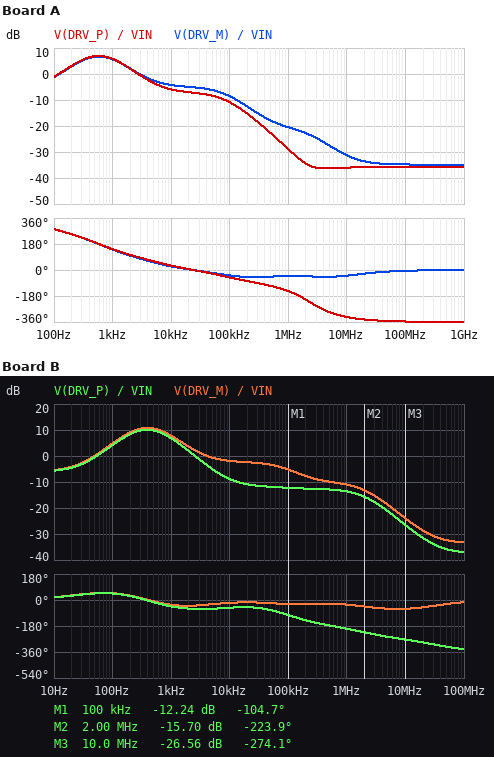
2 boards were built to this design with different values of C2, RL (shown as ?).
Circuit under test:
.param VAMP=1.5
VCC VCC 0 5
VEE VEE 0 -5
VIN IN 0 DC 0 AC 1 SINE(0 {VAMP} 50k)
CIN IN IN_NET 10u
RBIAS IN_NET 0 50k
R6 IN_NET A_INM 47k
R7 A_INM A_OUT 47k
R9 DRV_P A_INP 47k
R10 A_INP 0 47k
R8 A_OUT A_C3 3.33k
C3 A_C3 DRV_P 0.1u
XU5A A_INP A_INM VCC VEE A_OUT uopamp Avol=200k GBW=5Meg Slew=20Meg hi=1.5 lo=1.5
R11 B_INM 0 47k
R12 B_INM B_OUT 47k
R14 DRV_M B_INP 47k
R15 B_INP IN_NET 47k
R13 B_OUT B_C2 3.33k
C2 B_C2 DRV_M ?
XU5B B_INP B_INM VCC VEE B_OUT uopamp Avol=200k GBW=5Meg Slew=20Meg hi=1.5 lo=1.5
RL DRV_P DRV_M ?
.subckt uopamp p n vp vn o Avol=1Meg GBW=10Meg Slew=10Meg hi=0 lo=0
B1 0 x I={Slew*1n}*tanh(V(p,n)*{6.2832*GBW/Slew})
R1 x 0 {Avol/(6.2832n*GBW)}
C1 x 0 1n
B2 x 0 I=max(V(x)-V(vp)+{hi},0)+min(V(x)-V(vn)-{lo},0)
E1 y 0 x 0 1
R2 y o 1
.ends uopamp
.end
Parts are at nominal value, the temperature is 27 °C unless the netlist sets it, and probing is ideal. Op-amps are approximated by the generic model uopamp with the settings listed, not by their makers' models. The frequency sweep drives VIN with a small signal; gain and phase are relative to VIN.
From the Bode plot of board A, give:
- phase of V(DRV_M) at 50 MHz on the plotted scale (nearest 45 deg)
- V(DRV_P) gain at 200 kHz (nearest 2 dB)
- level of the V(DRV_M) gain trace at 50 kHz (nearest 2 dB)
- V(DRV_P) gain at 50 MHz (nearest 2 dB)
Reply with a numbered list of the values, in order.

1. 0 deg
2. -16 dB
3. -6 dB
4. -36 dB
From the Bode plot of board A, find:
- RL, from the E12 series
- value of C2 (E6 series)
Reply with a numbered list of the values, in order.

1. 390 Ω
2. 68 nF
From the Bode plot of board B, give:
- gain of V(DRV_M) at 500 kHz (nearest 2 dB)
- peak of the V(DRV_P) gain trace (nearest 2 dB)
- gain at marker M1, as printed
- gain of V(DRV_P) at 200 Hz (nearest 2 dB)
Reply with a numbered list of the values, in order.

1. -10 dB
2. 10 dB
3. -12.24 dB
4. 8 dB
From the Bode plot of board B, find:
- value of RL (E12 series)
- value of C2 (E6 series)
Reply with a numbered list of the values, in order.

1. 1.8 kΩ
2. 150 nF
